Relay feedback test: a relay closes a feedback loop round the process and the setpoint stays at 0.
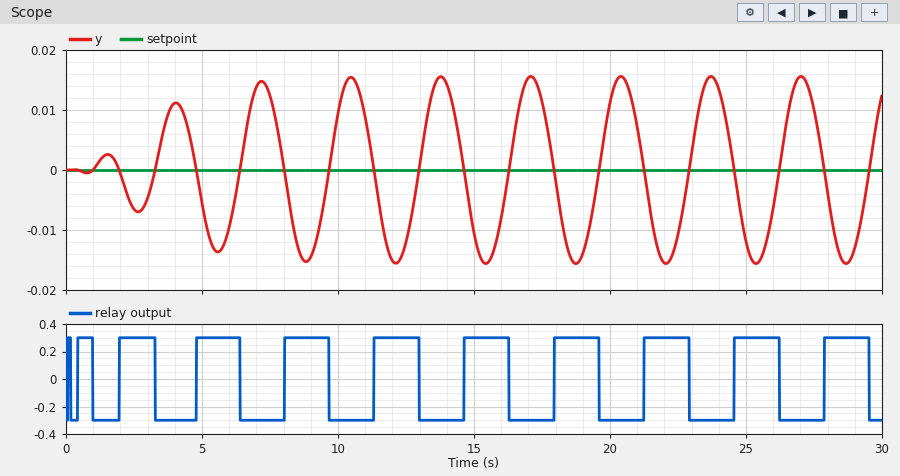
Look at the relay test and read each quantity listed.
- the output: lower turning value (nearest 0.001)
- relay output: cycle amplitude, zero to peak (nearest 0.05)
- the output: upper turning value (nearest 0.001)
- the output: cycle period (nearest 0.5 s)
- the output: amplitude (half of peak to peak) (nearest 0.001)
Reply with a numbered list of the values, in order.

1. -0.016
2. 0.30
3. 0.016
4. 3.5 s
5. 0.016
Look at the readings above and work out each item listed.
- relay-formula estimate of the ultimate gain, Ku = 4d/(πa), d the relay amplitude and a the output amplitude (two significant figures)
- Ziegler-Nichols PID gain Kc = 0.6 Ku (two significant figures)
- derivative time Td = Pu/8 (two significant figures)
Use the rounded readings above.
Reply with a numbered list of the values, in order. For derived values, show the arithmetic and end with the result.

1. 4 × 0.3 / (π × 0.016) = 24
2. 0.6 × 24 = 14
3. 3.5 / 8 = 0.44 s
